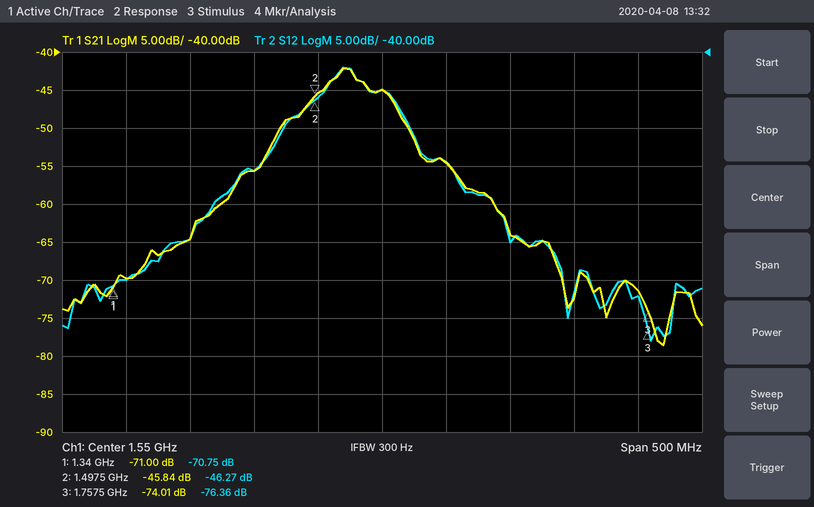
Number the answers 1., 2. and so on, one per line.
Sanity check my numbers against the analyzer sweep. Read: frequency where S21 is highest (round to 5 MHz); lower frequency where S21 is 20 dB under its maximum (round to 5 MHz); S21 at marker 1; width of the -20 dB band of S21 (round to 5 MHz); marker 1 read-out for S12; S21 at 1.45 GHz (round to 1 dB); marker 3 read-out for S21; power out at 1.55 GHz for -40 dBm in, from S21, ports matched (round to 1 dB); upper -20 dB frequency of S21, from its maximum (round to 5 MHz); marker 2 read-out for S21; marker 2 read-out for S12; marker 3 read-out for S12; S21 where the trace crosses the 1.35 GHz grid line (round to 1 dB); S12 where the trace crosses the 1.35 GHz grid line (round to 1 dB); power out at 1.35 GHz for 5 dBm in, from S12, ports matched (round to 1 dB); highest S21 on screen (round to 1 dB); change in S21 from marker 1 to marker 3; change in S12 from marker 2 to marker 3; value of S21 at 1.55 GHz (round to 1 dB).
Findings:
1. 1.520 GHz
2. 1.405 GHz
3. -71.00 dB
4. 240 MHz
5. -70.75 dB
6. -56 dB
7. -74.01 dB
8. -85 dBm
9. 1.645 GHz
10. -45.84 dB
11. -46.27 dB
12. -76.36 dB
13. -70 dB
14. -70 dB
15. -65 dBm
16. -42 dB
17. -3.01 dB
18. -30.09 dB
19. -45 dB
